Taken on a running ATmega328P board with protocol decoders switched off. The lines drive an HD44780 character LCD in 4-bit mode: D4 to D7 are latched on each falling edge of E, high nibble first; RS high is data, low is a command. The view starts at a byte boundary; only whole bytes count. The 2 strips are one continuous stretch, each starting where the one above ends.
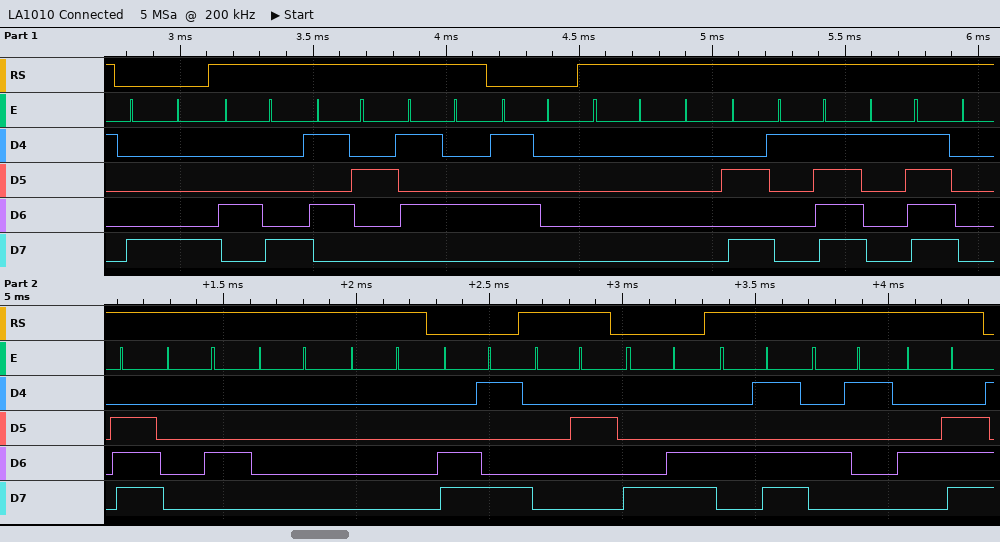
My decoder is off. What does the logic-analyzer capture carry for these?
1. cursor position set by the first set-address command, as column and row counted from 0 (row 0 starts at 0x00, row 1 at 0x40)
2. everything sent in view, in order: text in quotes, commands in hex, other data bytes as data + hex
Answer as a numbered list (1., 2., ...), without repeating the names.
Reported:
1. column 8, row 0
2. 0x88 "HRT" 0x50 data 00 0A 1F 1F 0E 04 00 00 0xC9 data 02 0x8C "MAN"
